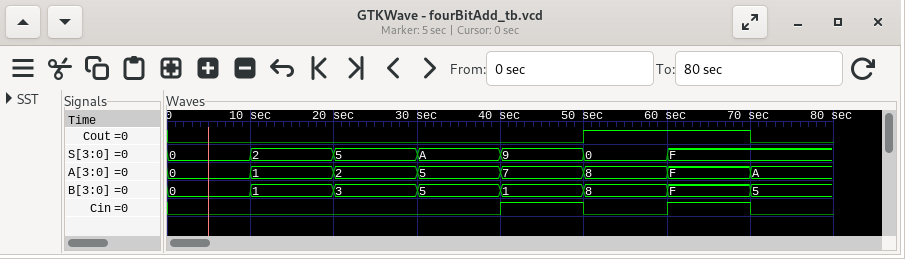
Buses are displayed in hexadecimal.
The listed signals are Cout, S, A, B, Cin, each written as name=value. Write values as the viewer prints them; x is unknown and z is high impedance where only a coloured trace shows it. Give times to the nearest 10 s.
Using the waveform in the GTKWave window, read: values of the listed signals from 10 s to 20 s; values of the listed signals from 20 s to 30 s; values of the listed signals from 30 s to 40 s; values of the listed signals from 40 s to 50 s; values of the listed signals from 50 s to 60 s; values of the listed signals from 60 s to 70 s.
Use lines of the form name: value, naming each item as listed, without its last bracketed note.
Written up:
values of the listed signals from 10 s to 20 s: Cout=0, S=2, A=1, B=1, Cin=0
values of the listed signals from 20 s to 30 s: Cout=0, S=5, A=2, B=3, Cin=0
values of the listed signals from 30 s to 40 s: Cout=0, S=A, A=5, B=5, Cin=0
values of the listed signals from 40 s to 50 s: Cout=0, S=9, A=7, B=1, Cin=1
values of the listed signals from 50 s to 60 s: Cout=1, S=0, A=8, B=8, Cin=0
values of the listed signals from 60 s to 70 s: Cout=1, S=F, A=F, B=F, Cin=1
